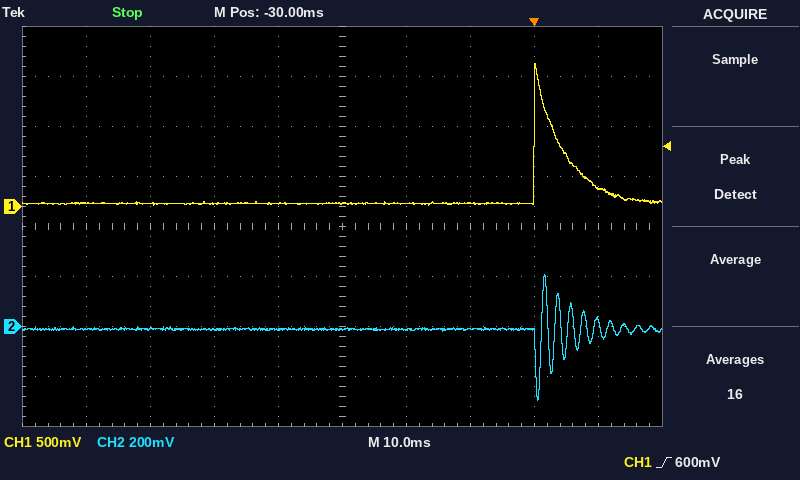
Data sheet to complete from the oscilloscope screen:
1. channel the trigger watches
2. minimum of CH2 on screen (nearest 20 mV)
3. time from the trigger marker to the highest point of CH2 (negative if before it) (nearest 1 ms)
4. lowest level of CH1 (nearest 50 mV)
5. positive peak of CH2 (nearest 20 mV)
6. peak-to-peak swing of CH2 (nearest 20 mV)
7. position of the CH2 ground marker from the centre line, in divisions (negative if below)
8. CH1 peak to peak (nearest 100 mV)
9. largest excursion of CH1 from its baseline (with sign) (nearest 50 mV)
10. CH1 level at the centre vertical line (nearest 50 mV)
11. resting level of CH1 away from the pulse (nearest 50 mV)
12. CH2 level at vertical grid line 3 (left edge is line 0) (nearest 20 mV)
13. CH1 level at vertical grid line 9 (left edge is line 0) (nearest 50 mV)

CH1
-300 mV
+2 ms
0 mV
200 mV
500 mV
-2.0 div
1.40 V
+1.40 V
50 mV
50 mV
-20 mV
200 mV
